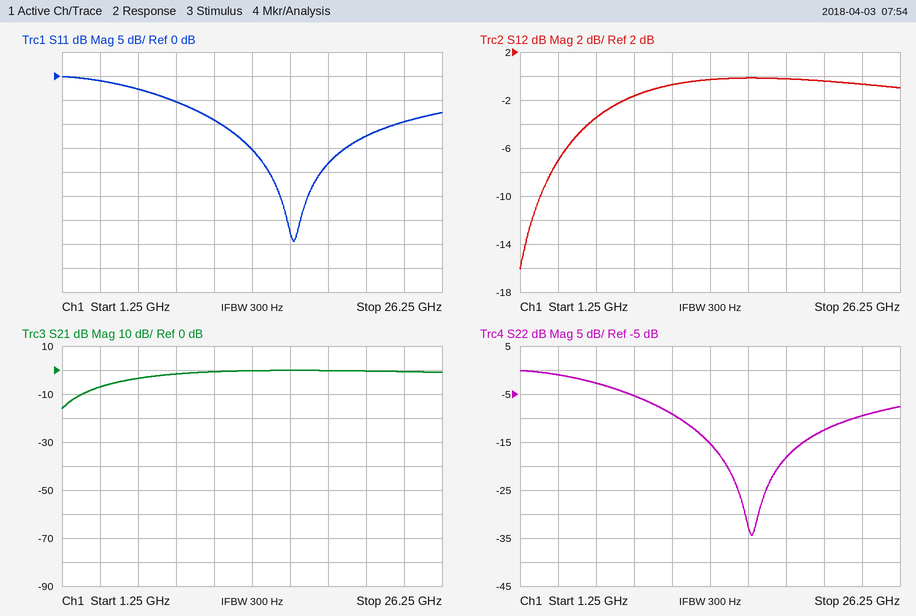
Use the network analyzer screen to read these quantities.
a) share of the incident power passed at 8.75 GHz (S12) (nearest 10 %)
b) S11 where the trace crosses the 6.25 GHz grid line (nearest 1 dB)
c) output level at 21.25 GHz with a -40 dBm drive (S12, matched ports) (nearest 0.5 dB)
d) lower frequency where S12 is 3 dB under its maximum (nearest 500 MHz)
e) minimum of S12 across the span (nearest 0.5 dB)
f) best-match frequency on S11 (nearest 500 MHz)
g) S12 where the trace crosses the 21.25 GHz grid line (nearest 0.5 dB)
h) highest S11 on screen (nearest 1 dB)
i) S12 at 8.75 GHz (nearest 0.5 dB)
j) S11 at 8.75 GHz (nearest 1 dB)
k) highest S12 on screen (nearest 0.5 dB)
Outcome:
70 %
-3 dB
-40.5 dBm
6.5 GHz
-16.0 dB
16.5 GHz
-0.5 dB
0 dB
-1.5 dB
-5 dB
0.0 dB
